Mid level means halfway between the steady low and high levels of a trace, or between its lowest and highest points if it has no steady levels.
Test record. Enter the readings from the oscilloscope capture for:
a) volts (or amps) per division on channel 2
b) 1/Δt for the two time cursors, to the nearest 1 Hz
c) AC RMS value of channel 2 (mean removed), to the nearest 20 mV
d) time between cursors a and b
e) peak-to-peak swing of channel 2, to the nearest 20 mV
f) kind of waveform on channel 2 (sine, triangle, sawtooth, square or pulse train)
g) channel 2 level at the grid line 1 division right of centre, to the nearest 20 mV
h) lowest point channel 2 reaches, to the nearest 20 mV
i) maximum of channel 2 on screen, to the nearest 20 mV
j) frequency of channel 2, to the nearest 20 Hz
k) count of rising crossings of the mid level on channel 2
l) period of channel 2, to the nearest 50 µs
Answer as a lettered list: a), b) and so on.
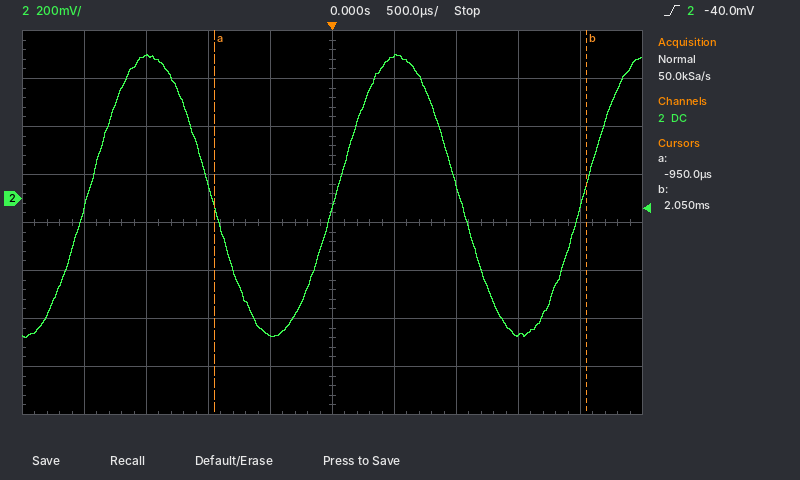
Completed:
a) 200 mV
b) 333 Hz
c) 420 mV
d) 3.00 ms
e) 1.18 V
f) sine
g) 600 mV
h) -580 mV
i) 600 mV
j) 500 Hz
k) 3
l) 2.00 ms
